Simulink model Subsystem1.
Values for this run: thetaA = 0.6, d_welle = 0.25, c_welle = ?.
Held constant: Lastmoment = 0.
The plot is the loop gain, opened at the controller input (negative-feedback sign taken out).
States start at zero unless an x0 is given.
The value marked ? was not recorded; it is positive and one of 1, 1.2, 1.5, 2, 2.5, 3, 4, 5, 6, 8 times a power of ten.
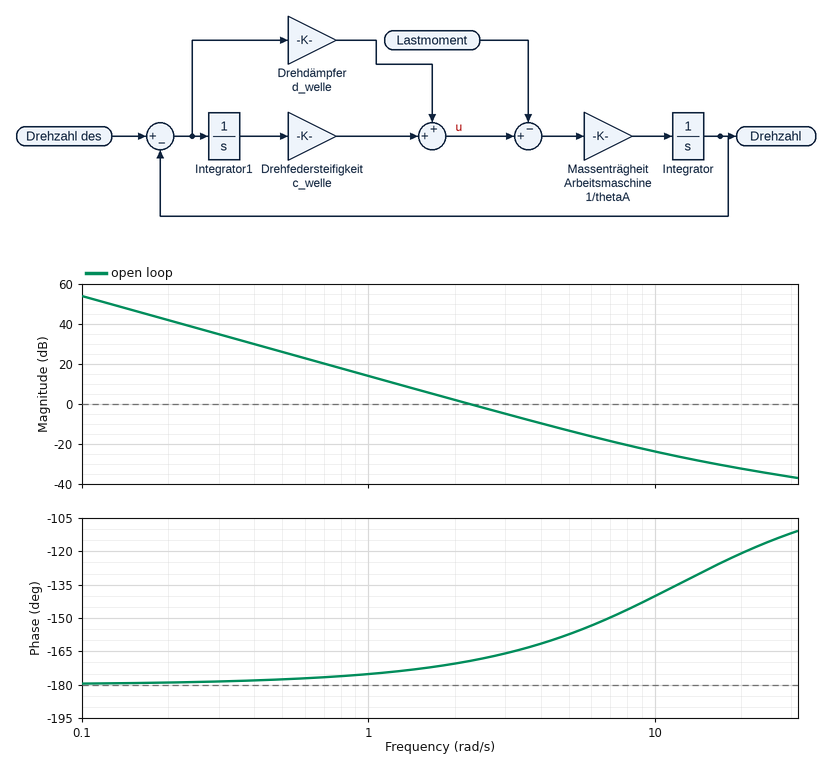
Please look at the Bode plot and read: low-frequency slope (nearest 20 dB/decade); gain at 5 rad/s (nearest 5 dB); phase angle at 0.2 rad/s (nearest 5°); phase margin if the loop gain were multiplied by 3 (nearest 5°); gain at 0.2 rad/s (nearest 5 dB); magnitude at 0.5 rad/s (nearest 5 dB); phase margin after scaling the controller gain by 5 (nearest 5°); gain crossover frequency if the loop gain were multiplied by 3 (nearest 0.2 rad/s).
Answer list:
-40 dB/decade
-15 dB
-180°
20°
40 dB
25 dB
25°
4.0 rad/s
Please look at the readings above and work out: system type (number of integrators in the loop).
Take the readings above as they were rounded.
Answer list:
2
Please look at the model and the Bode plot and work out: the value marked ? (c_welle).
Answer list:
3
